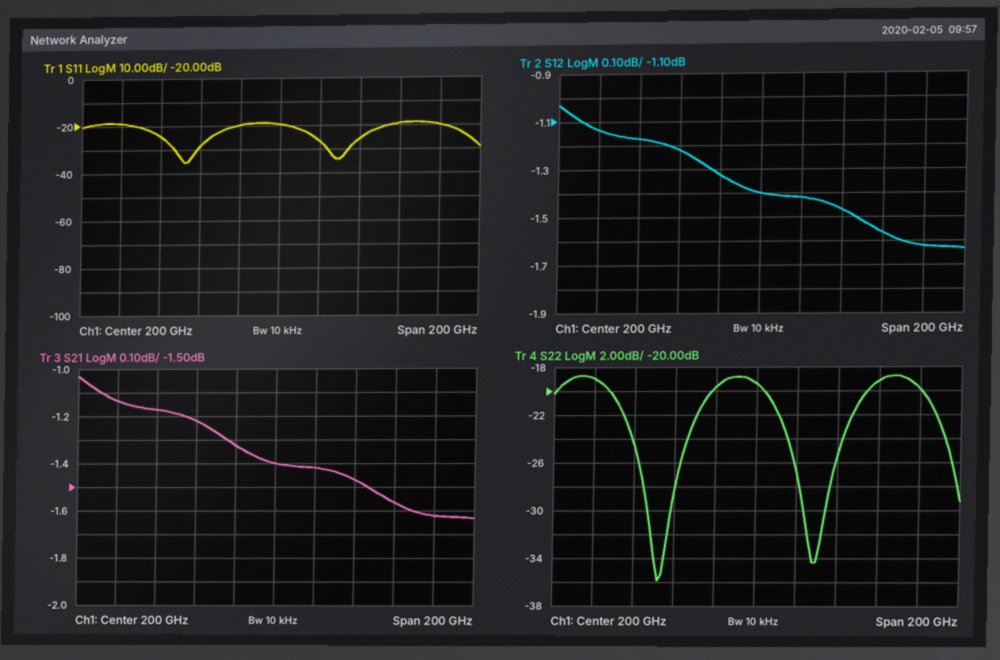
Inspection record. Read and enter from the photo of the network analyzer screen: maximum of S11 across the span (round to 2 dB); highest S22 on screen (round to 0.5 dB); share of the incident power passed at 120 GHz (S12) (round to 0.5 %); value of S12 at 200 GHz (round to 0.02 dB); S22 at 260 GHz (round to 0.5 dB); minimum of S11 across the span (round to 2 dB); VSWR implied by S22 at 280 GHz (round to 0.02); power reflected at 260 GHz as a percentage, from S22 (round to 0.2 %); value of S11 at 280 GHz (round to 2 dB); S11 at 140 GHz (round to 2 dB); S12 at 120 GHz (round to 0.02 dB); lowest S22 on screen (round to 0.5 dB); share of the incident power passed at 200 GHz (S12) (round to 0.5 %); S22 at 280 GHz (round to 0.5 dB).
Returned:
-18 dB
-18.5 dB
77.0 %
-1.40 dB
-19.0 dB
-36 dB
1.22
1.2 %
-20 dB
-24 dB
-1.14 dB
-36.0 dB
72.5 %
-20.0 dB
